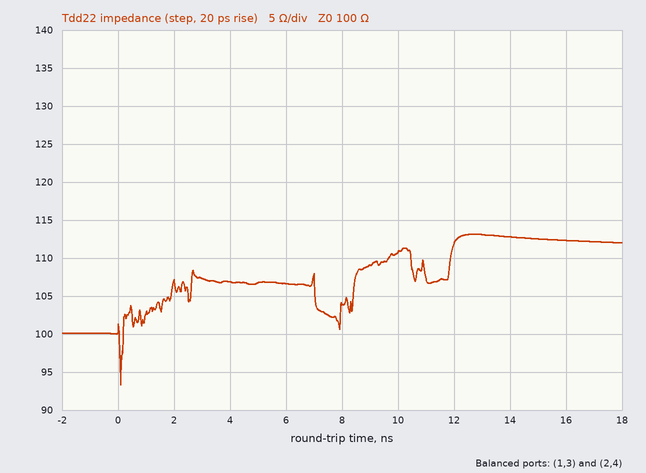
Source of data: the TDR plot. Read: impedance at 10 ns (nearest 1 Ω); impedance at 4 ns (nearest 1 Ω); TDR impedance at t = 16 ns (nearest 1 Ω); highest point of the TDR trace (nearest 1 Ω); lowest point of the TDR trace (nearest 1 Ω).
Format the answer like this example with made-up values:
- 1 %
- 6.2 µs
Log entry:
- 111 Ω
- 107 Ω
- 112 Ω
- 113 Ω
- 93 Ω
